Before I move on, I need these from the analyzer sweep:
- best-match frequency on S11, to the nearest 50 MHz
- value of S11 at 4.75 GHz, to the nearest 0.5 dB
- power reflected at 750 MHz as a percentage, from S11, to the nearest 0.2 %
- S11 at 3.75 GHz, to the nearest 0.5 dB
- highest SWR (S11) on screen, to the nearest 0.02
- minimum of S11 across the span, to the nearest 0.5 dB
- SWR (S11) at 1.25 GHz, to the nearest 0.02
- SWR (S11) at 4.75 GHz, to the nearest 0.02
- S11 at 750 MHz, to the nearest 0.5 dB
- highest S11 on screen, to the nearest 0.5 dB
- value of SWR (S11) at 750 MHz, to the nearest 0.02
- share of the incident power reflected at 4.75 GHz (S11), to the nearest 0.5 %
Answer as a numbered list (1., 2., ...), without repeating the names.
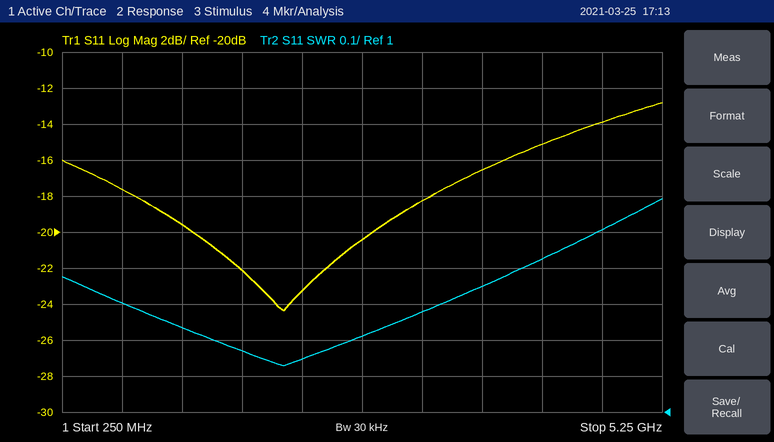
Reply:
1. 2.10 GHz
2. -14.0 dB
3. 1.8 %
4. -16.5 dB
5. 1.60
6. -24.5 dB
7. 1.24
8. 1.50
9. -17.5 dB
10. -13.0 dB
11. 1.30
12. 4.0 %
